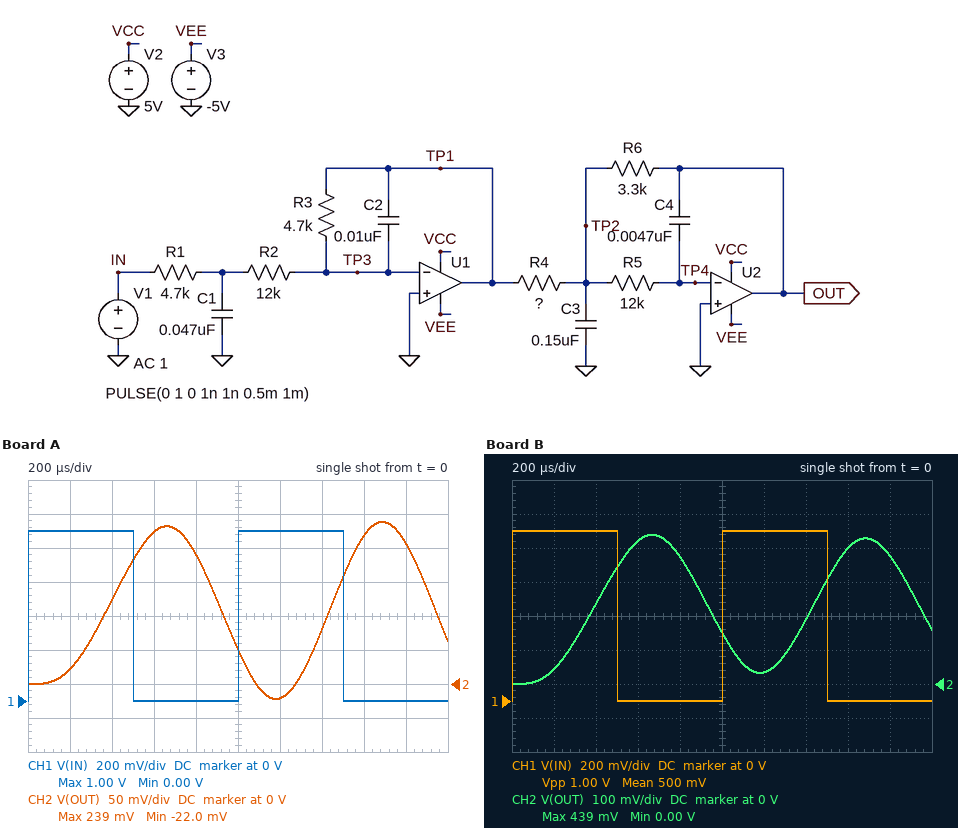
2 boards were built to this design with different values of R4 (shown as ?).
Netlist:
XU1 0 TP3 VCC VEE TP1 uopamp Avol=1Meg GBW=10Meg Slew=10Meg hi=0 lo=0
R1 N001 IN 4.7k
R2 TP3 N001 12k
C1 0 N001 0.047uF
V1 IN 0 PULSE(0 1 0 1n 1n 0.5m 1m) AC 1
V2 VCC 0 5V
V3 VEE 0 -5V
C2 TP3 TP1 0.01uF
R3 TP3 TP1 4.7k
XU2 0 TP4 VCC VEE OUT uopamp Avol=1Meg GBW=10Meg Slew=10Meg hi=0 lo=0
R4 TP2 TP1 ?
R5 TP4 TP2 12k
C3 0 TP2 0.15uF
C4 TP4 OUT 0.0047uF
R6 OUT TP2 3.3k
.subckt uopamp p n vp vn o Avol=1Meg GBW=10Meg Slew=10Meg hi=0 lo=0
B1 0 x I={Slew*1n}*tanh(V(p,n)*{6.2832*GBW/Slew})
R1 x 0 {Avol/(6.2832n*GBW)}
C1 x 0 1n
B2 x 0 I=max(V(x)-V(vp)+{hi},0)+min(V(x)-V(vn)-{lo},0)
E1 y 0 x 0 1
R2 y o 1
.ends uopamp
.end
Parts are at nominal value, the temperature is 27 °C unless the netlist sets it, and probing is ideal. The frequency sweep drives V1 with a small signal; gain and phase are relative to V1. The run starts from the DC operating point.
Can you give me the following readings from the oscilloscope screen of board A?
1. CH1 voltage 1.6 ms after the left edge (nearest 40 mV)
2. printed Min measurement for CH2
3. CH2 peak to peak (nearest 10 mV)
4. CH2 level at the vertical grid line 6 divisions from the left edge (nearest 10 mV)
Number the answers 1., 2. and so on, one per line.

1. 0 V
2. -22.0 mV
3. 260 mV
4. -20 mV
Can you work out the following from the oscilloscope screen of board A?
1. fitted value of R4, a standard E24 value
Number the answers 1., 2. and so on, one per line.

1. 4.3 kΩ
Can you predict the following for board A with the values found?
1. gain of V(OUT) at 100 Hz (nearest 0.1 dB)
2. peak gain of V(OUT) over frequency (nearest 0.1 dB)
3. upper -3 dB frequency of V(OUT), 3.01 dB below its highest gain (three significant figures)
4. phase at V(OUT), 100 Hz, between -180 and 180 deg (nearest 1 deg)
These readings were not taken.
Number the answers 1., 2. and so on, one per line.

1. -13.3 dB
2. -11.9 dB
3. 1.05 kHz
4. -12 deg
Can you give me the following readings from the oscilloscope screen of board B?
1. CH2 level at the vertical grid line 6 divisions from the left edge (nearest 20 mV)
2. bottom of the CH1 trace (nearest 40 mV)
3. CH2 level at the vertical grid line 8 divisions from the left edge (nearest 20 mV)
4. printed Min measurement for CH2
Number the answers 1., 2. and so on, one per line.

1. 40 mV
2. 0 V
3. 400 mV
4. 0.00 V
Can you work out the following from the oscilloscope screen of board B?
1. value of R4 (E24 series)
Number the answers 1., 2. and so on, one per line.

1. 2 kΩ
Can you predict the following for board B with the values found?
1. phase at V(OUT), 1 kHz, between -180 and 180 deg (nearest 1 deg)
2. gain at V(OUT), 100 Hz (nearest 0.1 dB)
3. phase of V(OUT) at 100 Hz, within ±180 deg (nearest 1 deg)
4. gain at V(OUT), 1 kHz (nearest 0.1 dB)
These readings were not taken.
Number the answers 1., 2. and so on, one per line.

1. -157 deg
2. -6.7 dB
3. -13 deg
4. -10.4 dB
